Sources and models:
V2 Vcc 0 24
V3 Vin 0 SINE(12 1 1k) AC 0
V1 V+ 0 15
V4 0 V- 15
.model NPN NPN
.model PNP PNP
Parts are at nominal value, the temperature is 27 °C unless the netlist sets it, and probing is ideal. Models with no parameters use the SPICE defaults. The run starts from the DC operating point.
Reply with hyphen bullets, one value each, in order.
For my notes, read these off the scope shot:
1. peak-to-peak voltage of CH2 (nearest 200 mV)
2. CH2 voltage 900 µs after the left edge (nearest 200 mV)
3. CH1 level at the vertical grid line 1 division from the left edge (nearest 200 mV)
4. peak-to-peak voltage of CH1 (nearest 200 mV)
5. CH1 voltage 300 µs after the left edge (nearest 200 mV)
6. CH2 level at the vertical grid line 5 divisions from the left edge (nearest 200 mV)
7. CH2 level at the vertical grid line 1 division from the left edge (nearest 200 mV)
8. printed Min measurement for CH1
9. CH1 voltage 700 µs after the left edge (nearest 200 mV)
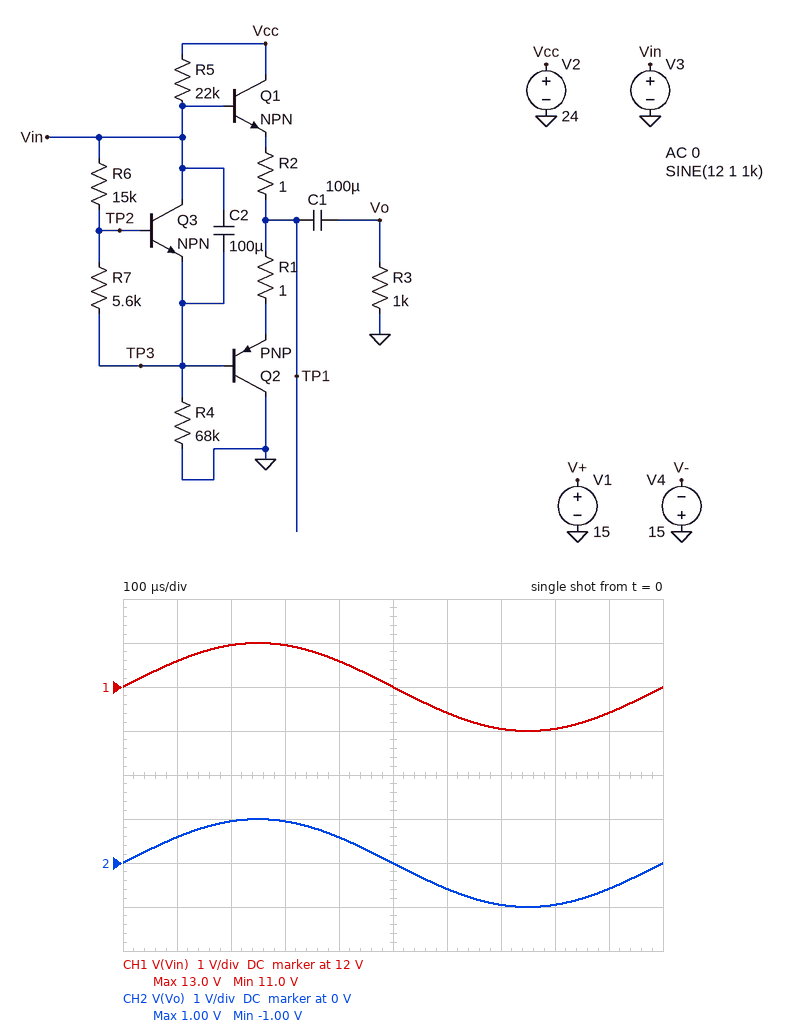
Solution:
- 2.0 V
- -600 mV
- 12.6 V
- 2.0 V
- 13.0 V
- 0 V
- 600 mV
- 11.0 V
- 11.0 V
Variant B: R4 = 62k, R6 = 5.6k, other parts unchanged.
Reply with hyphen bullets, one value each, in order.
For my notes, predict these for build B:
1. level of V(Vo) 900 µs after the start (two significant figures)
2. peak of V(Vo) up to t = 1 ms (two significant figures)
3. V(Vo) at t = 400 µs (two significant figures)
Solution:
- -530 mV
- 920 mV
- 520 mV
